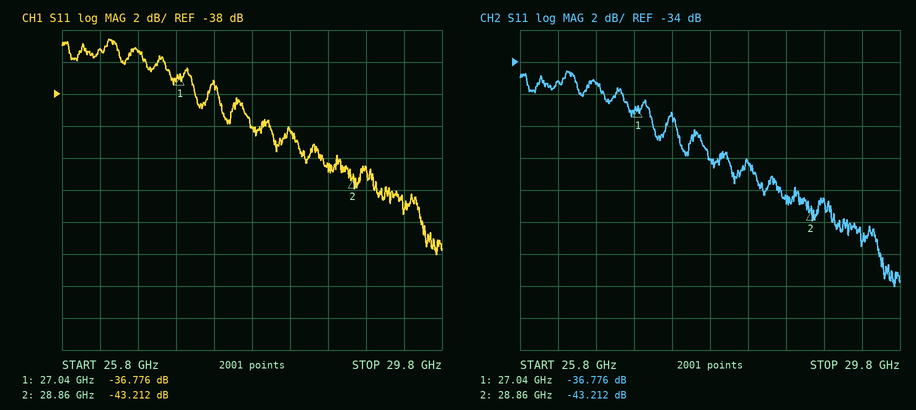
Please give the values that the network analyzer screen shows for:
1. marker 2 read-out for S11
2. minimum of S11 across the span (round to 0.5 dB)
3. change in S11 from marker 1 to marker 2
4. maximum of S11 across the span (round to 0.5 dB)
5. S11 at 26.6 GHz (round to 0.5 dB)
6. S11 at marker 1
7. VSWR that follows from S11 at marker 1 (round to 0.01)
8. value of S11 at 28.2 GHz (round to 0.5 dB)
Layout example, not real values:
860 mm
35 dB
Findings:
-43.212 dB
-48.0 dB
-6.436 dB
-34.5 dB
-35.5 dB
-36.776 dB
1.03
-40.5 dB
